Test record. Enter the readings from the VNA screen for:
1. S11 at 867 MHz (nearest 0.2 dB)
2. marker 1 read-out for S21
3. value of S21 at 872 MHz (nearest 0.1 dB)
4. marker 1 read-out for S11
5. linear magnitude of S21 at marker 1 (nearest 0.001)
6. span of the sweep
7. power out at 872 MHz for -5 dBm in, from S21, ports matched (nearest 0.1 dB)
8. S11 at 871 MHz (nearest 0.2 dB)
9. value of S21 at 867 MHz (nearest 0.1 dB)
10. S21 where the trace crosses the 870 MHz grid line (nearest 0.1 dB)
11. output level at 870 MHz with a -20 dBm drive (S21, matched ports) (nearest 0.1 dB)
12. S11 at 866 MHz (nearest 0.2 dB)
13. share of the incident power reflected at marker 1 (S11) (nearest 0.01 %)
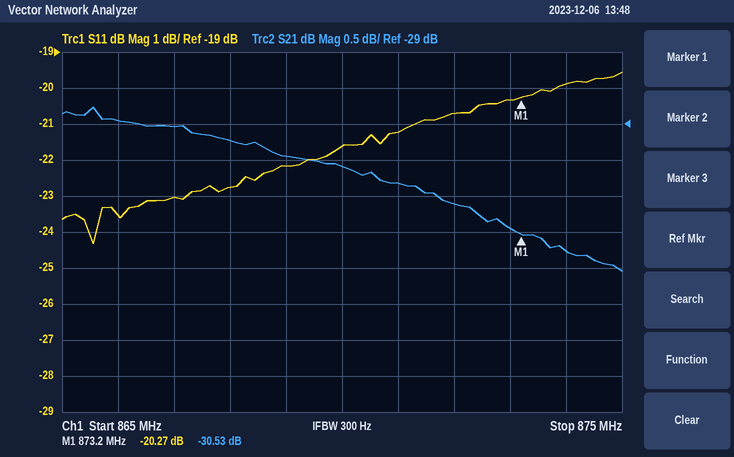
-23.0 dB
-30.53 dB
-30.1 dB
-20.27 dB
0.030
10 MHz
-35.1 dBm
-21.2 dB
-29.0 dB
-29.6 dB
-49.6 dBm
-23.6 dB
0.94 %
